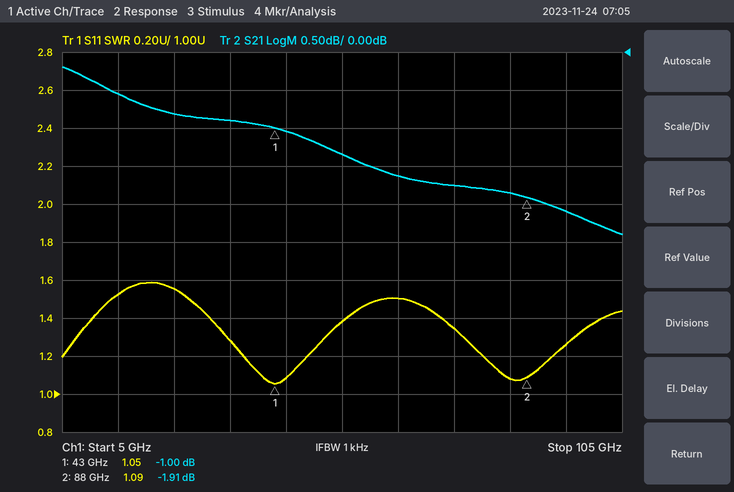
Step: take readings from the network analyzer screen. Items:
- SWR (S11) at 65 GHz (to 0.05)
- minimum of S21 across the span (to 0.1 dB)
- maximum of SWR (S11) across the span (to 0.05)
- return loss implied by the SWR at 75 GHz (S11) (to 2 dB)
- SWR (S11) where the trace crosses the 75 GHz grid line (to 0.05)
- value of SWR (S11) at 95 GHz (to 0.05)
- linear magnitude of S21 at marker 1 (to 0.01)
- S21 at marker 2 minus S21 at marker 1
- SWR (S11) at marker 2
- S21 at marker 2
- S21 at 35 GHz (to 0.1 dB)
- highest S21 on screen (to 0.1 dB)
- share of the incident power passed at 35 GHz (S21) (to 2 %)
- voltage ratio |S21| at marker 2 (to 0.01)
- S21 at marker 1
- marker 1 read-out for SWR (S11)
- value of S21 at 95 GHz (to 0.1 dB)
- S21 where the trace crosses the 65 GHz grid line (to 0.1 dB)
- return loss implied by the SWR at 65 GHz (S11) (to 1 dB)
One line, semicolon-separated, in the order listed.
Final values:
1.50; -2.4 dB; 1.60; 16 dB; 1.35; 1.25; 0.89; -0.91 dB; 1.09; -1.91 dB; -0.9 dB; -0.2 dB; 82 %; 0.80; -1.00 dB; 1.05; -2.1 dB; -1.6 dB; 14 dB
